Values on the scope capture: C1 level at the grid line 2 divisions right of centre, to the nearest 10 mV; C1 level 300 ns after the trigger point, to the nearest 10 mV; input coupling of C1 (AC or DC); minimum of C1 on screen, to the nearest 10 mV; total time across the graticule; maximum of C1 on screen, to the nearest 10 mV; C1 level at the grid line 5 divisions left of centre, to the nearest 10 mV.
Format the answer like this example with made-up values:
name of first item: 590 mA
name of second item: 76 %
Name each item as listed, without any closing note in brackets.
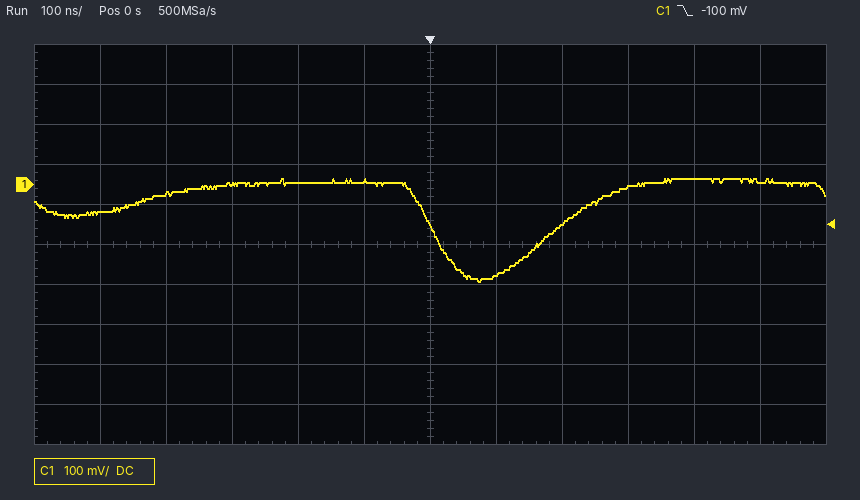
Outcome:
C1 level at the grid line 2 divisions right of centre, to the nearest 10 mV: -100 mV
C1 level 300 ns after the trigger point, to the nearest 10 mV: -10 mV
input coupling of C1: DC
minimum of C1 on screen, to the nearest 10 mV: -240 mV
total time across the graticule: 1.2 µs
maximum of C1 on screen, to the nearest 10 mV: 10 mV
C1 level at the grid line 5 divisions left of centre, to the nearest 10 mV: -70 mV
